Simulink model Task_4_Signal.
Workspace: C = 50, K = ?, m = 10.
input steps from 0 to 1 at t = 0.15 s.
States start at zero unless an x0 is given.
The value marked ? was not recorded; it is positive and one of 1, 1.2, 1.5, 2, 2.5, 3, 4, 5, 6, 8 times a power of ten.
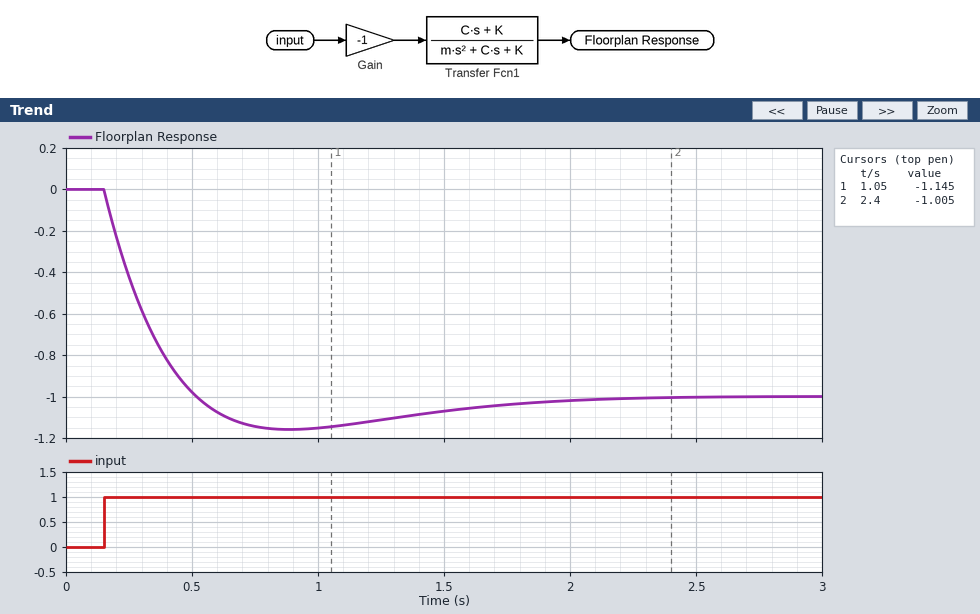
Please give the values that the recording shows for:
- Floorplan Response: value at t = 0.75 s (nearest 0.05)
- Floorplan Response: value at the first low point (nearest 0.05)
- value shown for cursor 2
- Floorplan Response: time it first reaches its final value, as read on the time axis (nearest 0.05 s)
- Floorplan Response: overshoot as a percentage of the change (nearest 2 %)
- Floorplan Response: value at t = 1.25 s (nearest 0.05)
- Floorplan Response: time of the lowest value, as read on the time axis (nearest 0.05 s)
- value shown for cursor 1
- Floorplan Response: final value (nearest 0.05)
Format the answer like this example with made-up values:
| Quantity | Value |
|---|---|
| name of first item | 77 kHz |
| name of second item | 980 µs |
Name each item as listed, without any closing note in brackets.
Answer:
| Quantity | Value |
|---|---|
| Floorplan Response: value at t = 0.75 s | -1.15 |
| Floorplan Response: value at the first low point | -1.15 |
| value shown for cursor 2 | -1.005 |
| Floorplan Response: time it first reaches its final value, as read on the time axis | 0.50 s |
| Floorplan Response: overshoot as a percentage of the change | 16 % |
| Floorplan Response: value at t = 1.25 s | -1.10 |
| Floorplan Response: time of the lowest value, as read on the time axis | 0.90 s |
| value shown for cursor 1 | -1.145 |
| Floorplan Response: final value | -1.00 |
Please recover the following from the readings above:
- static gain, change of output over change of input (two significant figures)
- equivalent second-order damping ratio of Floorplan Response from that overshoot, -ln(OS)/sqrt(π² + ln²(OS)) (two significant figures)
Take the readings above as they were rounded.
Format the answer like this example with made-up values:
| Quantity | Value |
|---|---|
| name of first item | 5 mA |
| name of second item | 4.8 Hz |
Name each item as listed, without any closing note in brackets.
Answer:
| Quantity | Value |
|---|---|
| static gain, change of output over change of input | -1.0 |
| equivalent second-order damping ratio of Floorplan Response from that overshoot, -ln(OS)/sqrt(π² + ln²(OS)) | 0.50 |
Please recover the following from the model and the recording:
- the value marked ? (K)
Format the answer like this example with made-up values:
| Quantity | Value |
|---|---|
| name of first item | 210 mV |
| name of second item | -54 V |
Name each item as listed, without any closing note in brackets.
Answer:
| Quantity | Value |
|---|---|
| the value marked ? | 80 |
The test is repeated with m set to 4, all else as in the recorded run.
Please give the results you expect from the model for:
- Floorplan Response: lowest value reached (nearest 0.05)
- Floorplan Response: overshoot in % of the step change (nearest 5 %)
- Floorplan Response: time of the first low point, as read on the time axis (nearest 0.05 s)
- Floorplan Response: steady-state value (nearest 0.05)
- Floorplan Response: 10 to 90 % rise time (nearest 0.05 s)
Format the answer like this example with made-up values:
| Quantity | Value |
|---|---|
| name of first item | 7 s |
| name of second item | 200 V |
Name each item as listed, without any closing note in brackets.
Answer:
| Quantity | Value |
|---|---|
| Floorplan Response: lowest value reached | -1.10 |
| Floorplan Response: overshoot in % of the step change | 10 % |
| Floorplan Response: time of the first low point, as read on the time axis | 0.55 s |
| Floorplan Response: steady-state value | -1.00 |
| Floorplan Response: 10 to 90 % rise time | 0.15 s |
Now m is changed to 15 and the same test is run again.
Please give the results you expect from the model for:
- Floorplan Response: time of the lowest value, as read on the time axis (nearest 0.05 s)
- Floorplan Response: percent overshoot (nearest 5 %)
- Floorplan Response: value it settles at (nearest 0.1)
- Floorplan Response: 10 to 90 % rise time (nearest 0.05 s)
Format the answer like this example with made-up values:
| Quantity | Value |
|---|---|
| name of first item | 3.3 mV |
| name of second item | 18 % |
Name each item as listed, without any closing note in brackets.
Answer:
| Quantity | Value |
|---|---|
| Floorplan Response: time of the lowest value, as read on the time axis | 1.10 s |
| Floorplan Response: percent overshoot | 20 % |
| Floorplan Response: value it settles at | -1.0 |
| Floorplan Response: 10 to 90 % rise time | 0.35 s |
